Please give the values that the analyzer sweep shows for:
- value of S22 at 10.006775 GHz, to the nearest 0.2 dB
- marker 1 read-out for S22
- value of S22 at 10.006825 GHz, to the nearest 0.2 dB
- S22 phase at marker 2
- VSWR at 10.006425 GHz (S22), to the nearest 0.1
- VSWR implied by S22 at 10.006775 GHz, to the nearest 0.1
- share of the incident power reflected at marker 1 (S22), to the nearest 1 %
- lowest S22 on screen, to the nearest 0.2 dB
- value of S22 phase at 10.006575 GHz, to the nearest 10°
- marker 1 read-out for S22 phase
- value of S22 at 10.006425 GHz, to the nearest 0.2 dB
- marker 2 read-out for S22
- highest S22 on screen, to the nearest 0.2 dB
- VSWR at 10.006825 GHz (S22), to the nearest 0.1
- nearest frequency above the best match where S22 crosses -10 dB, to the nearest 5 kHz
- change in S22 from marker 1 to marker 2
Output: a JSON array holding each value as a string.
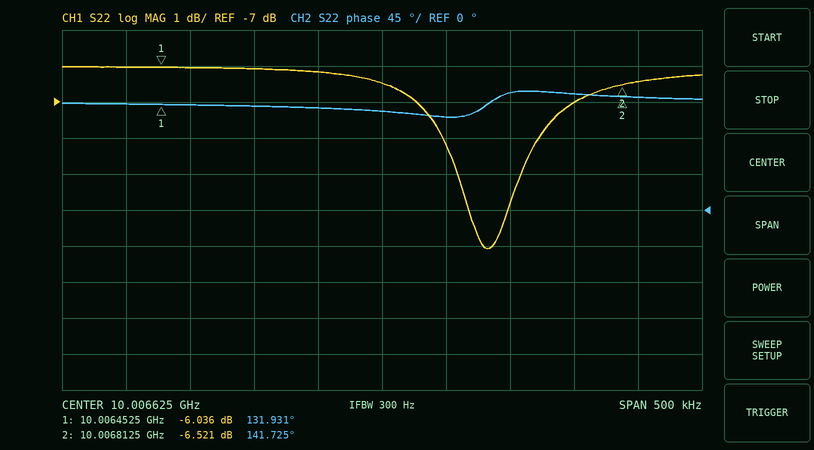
["-7.0 dB", "-6.036 dB", "-6.4 dB", "141.725°", "3.0", "2.6", "25 %", "-11.0 dB", "130°", "131.931°", "-6.0 dB", "-6.521 dB", "-6.0 dB", "2.8", "10.006725 GHz", "-0.485 dB"]
